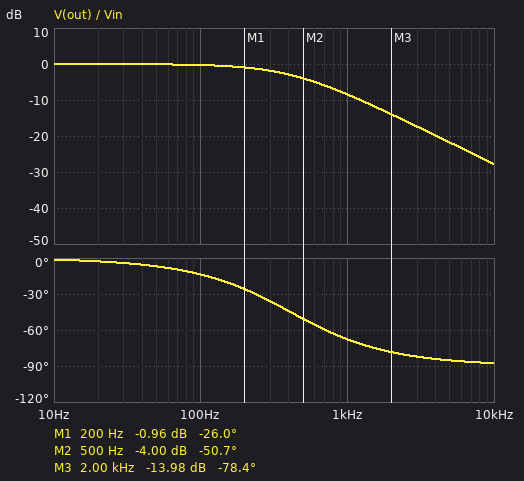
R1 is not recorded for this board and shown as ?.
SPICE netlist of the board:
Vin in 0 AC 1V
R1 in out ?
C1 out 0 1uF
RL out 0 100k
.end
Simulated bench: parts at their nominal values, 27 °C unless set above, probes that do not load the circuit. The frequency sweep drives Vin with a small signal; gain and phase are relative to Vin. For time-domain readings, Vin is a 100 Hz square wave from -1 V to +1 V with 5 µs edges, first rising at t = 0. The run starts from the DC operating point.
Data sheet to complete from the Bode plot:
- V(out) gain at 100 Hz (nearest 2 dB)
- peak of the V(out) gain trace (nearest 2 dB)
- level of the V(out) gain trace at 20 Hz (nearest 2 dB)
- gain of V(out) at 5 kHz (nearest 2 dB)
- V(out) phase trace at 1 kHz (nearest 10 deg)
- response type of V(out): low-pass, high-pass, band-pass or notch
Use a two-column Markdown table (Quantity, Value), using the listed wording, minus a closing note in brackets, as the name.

| Quantity | Value |
|---|---|
| V(out) gain at 100 Hz | 0 dB |
| peak of the V(out) gain trace | 0 dB |
| level of the V(out) gain trace at 20 Hz | 0 dB |
| gain of V(out) at 5 kHz | -22 dB |
| V(out) phase trace at 1 kHz | -70 deg |
| response type of V(out): low-pass, high-pass, band-pass or notch | low-pass |
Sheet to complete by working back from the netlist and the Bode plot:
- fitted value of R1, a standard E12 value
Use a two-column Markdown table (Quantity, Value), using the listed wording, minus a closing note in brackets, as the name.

| Quantity | Value |
|---|---|
| fitted value of R1, a standard E12 value | 390 Ω |
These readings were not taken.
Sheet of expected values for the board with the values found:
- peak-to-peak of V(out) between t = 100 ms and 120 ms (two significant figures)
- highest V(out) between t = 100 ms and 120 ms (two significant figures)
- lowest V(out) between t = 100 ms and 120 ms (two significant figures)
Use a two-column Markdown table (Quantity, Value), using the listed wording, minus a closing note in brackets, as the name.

| Quantity | Value |
|---|---|
| peak-to-peak of V(out) between t = 100 ms and 120 ms | 2.0 V |
| highest V(out) between t = 100 ms and 120 ms | 1.0 V |
| lowest V(out) between t = 100 ms and 120 ms | -1.0 V |
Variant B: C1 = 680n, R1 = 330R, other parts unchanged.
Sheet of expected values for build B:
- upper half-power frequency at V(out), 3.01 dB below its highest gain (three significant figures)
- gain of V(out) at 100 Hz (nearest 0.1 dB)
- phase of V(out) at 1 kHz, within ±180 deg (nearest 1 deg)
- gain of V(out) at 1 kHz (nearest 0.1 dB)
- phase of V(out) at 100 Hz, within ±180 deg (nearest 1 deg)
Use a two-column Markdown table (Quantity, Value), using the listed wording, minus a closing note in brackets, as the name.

| Quantity | Value |
|---|---|
| upper half-power frequency at V(out), 3.01 dB below its highest gain | 712 Hz |
| gain of V(out) at 100 Hz | -0.1 dB |
| phase of V(out) at 1 kHz, within ±180 deg | -55 deg |
| gain of V(out) at 1 kHz | -4.8 dB |
| phase of V(out) at 100 Hz, within ±180 deg | -8 deg |
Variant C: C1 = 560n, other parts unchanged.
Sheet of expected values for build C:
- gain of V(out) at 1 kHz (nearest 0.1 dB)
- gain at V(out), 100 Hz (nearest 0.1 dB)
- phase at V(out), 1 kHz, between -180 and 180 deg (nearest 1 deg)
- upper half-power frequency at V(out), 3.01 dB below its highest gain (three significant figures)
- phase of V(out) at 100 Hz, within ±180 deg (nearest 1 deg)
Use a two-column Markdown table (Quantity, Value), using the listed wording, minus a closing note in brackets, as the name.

| Quantity | Value |
|---|---|
| gain of V(out) at 1 kHz | -4.6 dB |
| gain at V(out), 100 Hz | -0.1 dB |
| phase at V(out), 1 kHz, between -180 and 180 deg | -54 deg |
| upper half-power frequency at V(out), 3.01 dB below its highest gain | 732 Hz |
| phase of V(out) at 100 Hz, within ±180 deg | -8 deg |
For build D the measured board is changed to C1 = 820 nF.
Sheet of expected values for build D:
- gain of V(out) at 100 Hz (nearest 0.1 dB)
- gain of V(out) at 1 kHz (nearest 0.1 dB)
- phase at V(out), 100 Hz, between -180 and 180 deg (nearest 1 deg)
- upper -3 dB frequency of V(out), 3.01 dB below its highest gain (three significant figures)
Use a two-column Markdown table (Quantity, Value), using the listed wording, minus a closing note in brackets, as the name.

| Quantity | Value |
|---|---|
| gain of V(out) at 100 Hz | -0.2 dB |
| gain of V(out) at 1 kHz | -7.0 dB |
| phase at V(out), 100 Hz, between -180 and 180 deg | -11 deg |
| upper -3 dB frequency of V(out), 3.01 dB below its highest gain | 500 Hz |
